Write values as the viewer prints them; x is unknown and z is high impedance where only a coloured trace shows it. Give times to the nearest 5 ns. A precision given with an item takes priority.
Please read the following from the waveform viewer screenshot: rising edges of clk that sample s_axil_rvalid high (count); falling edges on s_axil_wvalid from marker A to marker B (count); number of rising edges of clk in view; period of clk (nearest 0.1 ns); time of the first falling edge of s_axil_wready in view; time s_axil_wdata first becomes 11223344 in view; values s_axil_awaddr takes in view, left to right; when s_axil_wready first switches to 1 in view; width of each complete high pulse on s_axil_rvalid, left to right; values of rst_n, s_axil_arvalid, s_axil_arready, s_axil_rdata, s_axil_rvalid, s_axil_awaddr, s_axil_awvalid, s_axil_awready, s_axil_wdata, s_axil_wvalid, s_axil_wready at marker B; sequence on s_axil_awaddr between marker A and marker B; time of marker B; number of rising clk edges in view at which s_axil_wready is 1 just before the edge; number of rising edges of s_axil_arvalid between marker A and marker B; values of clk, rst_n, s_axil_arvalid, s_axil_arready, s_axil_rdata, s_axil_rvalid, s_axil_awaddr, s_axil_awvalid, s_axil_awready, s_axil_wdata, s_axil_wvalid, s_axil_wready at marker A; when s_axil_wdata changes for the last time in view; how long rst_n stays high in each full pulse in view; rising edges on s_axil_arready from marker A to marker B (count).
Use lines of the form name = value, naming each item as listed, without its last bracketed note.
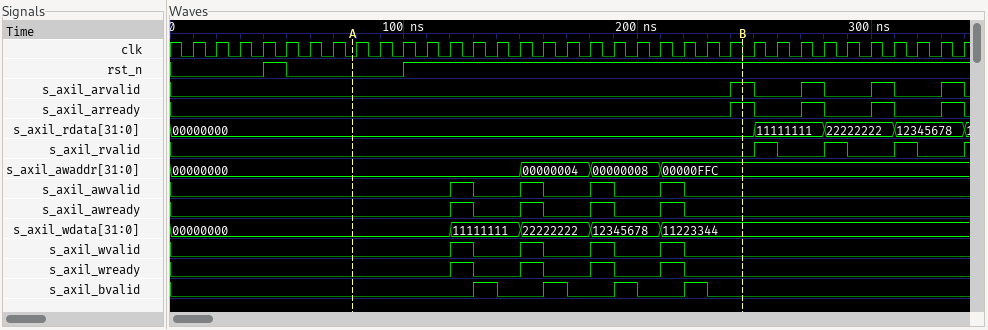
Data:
rising edges of clk that sample s_axil_rvalid high = 3
falling edges on s_axil_wvalid from marker A to marker B = 4
number of rising edges of clk in view = 34
period of clk = 10 ns
time of the first falling edge of s_axil_wready in view = 130 ns
time s_axil_wdata first becomes 11223344 in view = 210 ns
values s_axil_awaddr takes in view, left to right = 00000000, 00000004, 00000008, 00000FFC
when s_axil_wready first switches to 1 in view = 120 ns
width of each complete high pulse on s_axil_rvalid, left to right = 10 ns, 10 ns, 10 ns
values of rst_n, s_axil_arvalid, s_axil_arready, s_axil_rdata, s_axil_rvalid, s_axil_awaddr, s_axil_awvalid, s_axil_awready, s_axil_wdata, s_axil_wvalid, s_axil_wready at marker B = rst_n=1, s_axil_arvalid=1, s_axil_arready=1, s_axil_rdata=00000000, s_axil_rvalid=0, s_axil_awaddr=00000FFC, s_axil_awvalid=0, s_axil_awready=0, s_axil_wdata=11223344, s_axil_wvalid=0, s_axil_wready=0
sequence on s_axil_awaddr between marker A and marker B = 00000000, 00000004, 00000008, 00000FFC
time of marker B = 245 ns
number of rising clk edges in view at which s_axil_wready is 1 just before the edge = 4
number of rising edges of s_axil_arvalid between marker A and marker B = 1
values of clk, rst_n, s_axil_arvalid, s_axil_arready, s_axil_rdata, s_axil_rvalid, s_axil_awaddr, s_axil_awvalid, s_axil_awready, s_axil_wdata, s_axil_wvalid, s_axil_wready at marker A = clk=0, rst_n=0, s_axil_arvalid=0, s_axil_arready=0, s_axil_rdata=00000000, s_axil_rvalid=0, s_axil_awaddr=00000000, s_axil_awvalid=0, s_axil_awready=0, s_axil_wdata=00000000, s_axil_wvalid=0, s_axil_wready=0
when s_axil_wdata changes for the last time in view = 210 ns
how long rst_n stays high in each full pulse in view = 10 ns
rising edges on s_axil_arready from marker A to marker B = 1
